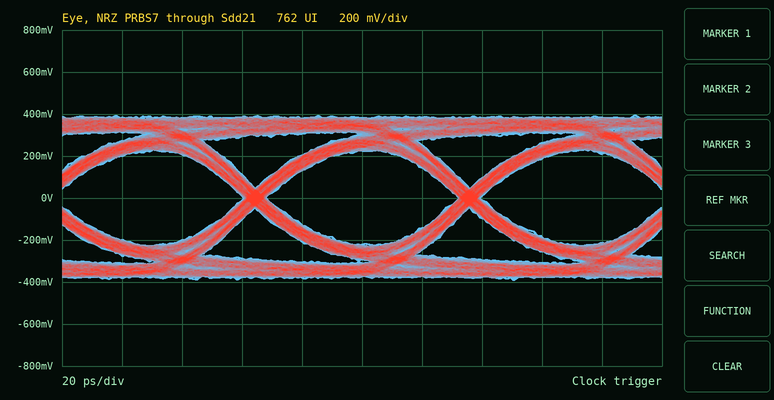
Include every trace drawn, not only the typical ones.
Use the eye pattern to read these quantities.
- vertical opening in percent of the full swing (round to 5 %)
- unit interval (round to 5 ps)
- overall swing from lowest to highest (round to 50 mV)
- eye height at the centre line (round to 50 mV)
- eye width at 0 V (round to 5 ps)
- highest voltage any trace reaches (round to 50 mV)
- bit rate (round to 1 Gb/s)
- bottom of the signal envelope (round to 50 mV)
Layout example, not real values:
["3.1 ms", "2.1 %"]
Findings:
["55 %", "70 ps", "800 mV", "450 mV", "65 ps", "400 mV", "14 Gb/s", "-400 mV"]
